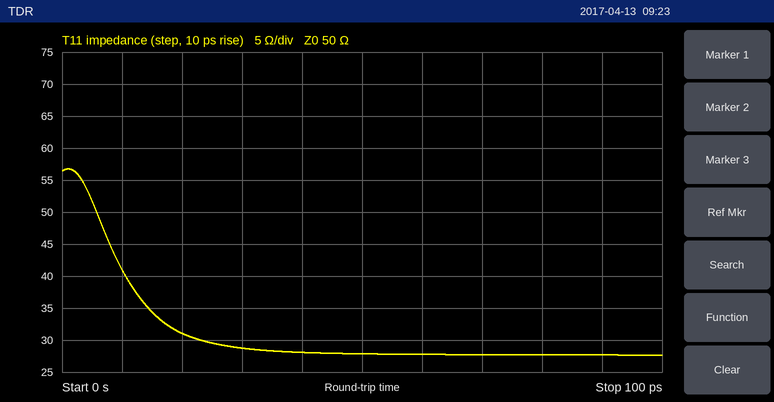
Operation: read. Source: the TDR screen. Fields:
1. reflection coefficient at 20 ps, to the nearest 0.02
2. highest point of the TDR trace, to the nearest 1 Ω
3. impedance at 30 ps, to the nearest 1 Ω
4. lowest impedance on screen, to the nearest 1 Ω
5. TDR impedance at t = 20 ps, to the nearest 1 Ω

-0.24
57 Ω
29 Ω
28 Ω
31 Ω
